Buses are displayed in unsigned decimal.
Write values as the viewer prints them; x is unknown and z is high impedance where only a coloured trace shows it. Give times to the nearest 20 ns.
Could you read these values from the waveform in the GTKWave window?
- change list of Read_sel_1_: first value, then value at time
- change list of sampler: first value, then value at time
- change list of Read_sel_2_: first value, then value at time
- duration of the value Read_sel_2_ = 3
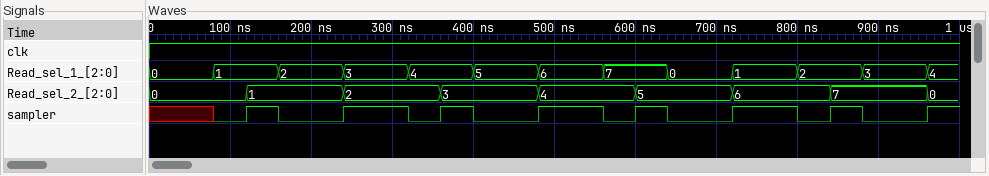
0, 1 at 80 ns, 2 at 160 ns, 3 at 240 ns, 4 at 320 ns, 5 at 400 ns, 6 at 480 ns, 7 at 560 ns, 0 at 640 ns, 1 at 720 ns, 2 at 800 ns, 3 at 880 ns, 4 at 960 ns
x, 0 at 80 ns, 1 at 120 ns, 0 at 160 ns, 1 at 240 ns, 0 at 320 ns, 1 at 360 ns, 0 at 400 ns, 1 at 480 ns, 0 at 560 ns, 1 at 600 ns, 0 at 640 ns, 1 at 720 ns, 0 at 800 ns, 1 at 840 ns, 0 at 880 ns, 1 at 960 ns
0, 1 at 120 ns, 2 at 240 ns, 3 at 360 ns, 4 at 480 ns, 5 at 600 ns, 6 at 720 ns, 7 at 840 ns, 0 at 960 ns
120 ns
